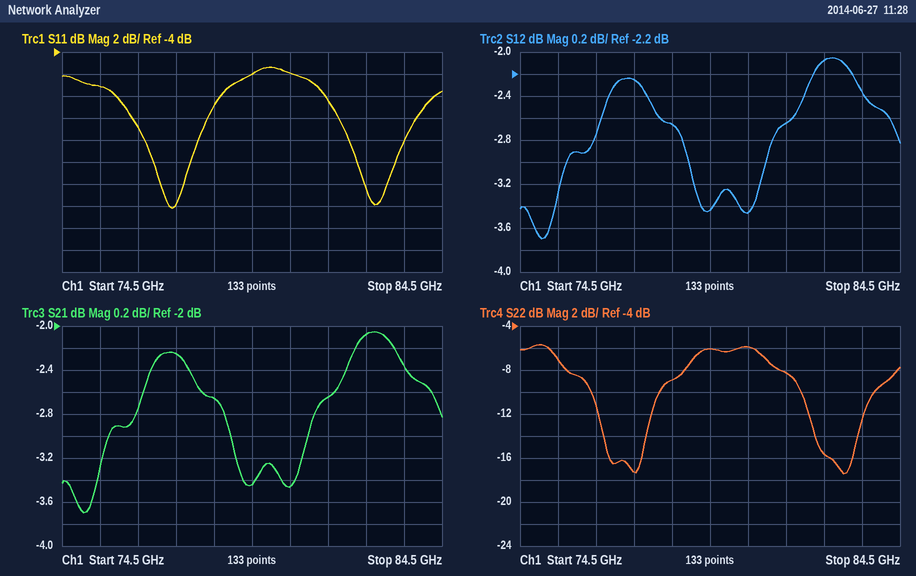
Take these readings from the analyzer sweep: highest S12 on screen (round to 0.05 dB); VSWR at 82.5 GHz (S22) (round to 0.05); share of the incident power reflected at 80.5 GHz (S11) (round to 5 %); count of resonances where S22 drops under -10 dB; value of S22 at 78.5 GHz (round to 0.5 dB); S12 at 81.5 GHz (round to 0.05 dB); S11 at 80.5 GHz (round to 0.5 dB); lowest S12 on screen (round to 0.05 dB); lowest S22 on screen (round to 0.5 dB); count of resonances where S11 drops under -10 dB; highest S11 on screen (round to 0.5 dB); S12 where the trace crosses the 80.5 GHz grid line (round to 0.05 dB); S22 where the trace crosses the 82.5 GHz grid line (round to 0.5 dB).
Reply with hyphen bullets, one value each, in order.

- -2.05 dB
- 1.40
- 25 %
- 2
- -9.0 dB
- -2.65 dB
- -6.0 dB
- -3.70 dB
- -17.5 dB
- 2
- -5.5 dB
- -3.45 dB
- -15.5 dB
